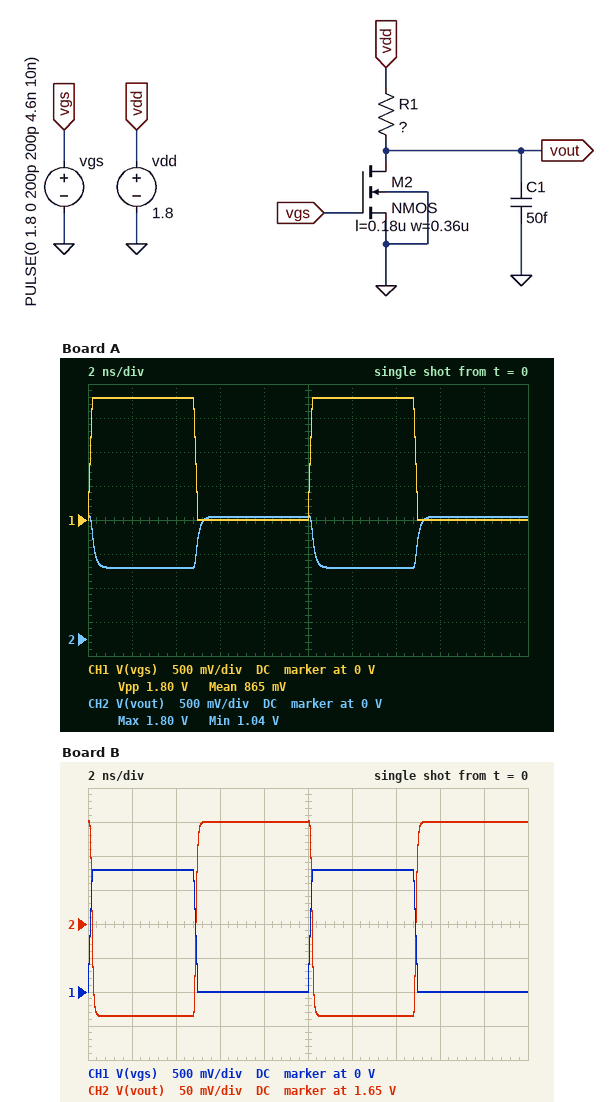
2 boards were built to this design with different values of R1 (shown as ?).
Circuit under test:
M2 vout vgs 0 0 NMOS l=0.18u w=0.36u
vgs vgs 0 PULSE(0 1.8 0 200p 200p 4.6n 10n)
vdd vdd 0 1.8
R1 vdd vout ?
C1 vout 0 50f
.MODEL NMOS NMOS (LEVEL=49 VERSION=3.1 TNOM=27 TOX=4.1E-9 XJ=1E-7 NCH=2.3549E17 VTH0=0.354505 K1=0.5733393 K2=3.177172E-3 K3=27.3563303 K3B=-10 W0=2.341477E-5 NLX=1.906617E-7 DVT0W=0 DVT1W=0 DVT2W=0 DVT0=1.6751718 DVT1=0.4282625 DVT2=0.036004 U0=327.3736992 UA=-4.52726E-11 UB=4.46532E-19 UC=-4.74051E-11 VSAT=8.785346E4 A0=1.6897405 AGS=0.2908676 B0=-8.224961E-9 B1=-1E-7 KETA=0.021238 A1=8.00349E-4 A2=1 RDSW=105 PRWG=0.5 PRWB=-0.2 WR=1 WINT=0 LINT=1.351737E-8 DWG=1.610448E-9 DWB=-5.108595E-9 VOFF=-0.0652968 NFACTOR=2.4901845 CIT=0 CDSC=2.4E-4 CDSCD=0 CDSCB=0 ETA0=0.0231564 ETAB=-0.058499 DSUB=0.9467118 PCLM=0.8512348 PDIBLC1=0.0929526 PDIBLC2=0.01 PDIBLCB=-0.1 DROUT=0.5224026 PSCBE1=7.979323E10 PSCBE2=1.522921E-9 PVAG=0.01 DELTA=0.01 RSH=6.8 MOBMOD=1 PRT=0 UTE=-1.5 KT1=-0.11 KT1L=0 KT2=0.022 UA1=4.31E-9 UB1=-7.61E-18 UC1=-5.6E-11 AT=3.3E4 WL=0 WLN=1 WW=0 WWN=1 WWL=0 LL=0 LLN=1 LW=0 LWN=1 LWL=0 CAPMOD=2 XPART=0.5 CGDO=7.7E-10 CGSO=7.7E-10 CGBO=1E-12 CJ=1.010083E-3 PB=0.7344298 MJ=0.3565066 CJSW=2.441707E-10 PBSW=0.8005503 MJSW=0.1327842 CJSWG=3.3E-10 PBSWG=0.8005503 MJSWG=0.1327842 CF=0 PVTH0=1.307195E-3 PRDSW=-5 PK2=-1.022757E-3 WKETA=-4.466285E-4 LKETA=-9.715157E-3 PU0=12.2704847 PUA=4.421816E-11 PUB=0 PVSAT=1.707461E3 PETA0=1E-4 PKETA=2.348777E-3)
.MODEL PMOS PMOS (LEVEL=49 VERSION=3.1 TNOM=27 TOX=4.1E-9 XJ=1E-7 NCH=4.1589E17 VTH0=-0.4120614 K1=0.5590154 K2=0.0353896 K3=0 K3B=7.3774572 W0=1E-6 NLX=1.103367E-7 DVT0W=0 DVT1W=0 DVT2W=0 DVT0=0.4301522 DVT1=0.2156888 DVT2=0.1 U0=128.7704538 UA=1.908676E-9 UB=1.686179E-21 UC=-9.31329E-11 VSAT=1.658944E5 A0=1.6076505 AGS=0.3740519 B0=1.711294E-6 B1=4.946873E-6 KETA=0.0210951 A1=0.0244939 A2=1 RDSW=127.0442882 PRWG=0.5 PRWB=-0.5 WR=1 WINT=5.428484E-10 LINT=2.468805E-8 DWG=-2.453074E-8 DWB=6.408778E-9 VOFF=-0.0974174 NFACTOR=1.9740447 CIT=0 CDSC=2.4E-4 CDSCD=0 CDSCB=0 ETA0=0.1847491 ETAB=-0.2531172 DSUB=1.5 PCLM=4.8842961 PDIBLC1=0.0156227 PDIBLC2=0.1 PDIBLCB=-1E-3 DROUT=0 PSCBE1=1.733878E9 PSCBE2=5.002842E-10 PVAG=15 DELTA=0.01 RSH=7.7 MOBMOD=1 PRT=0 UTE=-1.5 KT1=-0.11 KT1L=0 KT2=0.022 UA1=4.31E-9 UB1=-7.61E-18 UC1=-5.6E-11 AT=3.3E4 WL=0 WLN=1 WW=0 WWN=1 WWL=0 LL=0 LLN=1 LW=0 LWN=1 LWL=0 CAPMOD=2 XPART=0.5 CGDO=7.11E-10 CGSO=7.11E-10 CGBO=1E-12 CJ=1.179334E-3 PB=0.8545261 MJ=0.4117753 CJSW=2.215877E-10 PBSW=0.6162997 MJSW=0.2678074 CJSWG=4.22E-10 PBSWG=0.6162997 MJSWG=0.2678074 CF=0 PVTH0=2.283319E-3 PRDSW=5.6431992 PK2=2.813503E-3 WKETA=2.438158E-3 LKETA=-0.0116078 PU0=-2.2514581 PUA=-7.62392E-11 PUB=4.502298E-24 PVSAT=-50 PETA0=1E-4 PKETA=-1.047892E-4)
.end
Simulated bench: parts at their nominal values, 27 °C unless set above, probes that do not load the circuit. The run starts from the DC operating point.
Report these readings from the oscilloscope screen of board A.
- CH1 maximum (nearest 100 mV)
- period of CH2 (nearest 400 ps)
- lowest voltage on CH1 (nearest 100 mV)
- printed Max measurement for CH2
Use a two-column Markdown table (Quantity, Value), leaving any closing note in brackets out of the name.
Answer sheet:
| Quantity | Value |
|---|---|
| CH1 maximum | 1.8 V |
| period of CH2 | 10.0 ns |
| lowest voltage on CH1 | 0 V |
| printed Max measurement for CH2 | 1.80 V |
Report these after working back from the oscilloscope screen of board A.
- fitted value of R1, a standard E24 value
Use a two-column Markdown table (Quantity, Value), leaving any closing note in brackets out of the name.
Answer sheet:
| Quantity | Value |
|---|---|
| fitted value of R1, a standard E24 value | 3 kΩ |
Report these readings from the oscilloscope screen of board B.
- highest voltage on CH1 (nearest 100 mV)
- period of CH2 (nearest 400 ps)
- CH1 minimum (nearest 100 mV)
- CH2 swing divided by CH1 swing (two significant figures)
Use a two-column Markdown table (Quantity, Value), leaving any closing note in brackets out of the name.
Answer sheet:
| Quantity | Value |
|---|---|
| highest voltage on CH1 | 1.8 V |
| period of CH2 | 10.0 ns |
| CH1 minimum | 0 V |
| CH2 swing divided by CH1 swing | 0.16 |
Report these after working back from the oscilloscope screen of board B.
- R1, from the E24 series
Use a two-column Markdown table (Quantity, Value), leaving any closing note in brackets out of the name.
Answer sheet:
| Quantity | Value |
|---|---|
| R1, from the E24 series | 1.1 kΩ |
